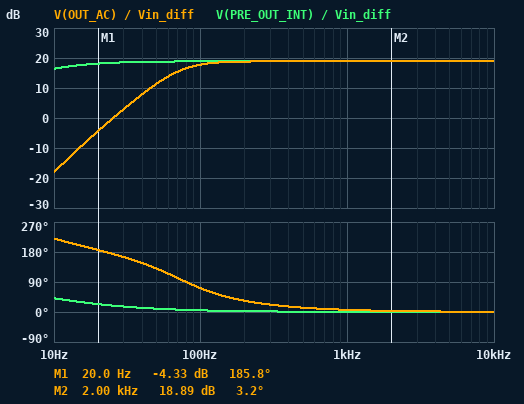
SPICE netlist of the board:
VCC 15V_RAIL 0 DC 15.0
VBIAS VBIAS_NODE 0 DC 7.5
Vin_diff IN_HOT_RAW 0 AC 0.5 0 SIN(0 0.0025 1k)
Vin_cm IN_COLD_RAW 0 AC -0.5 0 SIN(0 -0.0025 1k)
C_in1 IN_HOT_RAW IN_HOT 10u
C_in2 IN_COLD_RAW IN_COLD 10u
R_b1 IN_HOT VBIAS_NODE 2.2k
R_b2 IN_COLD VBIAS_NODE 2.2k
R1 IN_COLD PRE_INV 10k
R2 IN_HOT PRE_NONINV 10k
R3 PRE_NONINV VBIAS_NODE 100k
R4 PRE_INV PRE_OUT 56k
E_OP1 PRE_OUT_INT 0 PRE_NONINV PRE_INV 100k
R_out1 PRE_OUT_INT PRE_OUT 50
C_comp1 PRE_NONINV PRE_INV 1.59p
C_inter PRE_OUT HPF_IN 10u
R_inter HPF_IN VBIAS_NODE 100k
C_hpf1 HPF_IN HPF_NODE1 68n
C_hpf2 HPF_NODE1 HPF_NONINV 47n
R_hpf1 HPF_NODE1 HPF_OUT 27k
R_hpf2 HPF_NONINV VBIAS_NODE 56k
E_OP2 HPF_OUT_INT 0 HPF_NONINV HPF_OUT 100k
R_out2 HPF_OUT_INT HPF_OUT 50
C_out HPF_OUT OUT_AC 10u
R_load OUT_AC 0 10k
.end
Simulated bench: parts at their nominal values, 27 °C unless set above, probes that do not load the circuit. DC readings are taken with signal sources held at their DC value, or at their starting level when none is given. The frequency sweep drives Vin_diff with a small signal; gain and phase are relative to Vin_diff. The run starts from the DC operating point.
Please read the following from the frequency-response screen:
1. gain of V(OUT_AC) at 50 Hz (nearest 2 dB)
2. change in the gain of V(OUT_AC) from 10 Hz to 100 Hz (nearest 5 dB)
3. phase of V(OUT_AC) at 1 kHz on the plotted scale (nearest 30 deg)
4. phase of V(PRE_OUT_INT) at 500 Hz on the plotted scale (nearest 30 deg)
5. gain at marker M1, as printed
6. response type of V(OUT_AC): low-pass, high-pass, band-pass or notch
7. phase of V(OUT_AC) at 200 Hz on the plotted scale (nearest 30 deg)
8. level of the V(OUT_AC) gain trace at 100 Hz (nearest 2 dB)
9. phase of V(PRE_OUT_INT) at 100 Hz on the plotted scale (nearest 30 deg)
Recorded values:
12 dB
35 dB
0 deg
0 deg
-4.33 dB
high-pass
30 deg
18 dB
0 deg
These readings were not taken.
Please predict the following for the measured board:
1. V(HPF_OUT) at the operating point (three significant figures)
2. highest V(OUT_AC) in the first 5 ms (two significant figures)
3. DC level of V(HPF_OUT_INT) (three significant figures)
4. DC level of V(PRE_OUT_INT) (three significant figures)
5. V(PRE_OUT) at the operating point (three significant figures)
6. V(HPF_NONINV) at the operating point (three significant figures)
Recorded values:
7.50 V
29 mV
7.50 V
7.50 V
7.50 V
7.50 V
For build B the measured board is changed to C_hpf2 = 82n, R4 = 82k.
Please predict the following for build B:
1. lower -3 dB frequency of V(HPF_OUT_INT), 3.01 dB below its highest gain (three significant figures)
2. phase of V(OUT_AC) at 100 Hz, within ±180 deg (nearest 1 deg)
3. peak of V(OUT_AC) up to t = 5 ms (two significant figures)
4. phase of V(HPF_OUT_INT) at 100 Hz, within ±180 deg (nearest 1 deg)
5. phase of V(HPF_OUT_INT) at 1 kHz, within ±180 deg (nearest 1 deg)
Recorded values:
55.0 Hz
54 deg
41 mV
53 deg
5 deg
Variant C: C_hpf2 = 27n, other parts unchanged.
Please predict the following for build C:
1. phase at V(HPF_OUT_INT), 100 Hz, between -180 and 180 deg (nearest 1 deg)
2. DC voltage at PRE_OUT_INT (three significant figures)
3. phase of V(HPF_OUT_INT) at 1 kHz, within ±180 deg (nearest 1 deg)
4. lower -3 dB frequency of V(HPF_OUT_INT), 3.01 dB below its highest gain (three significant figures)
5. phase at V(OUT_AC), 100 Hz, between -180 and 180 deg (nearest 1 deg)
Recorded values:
92 deg
7.50 V
9 deg
105 Hz
93 deg
